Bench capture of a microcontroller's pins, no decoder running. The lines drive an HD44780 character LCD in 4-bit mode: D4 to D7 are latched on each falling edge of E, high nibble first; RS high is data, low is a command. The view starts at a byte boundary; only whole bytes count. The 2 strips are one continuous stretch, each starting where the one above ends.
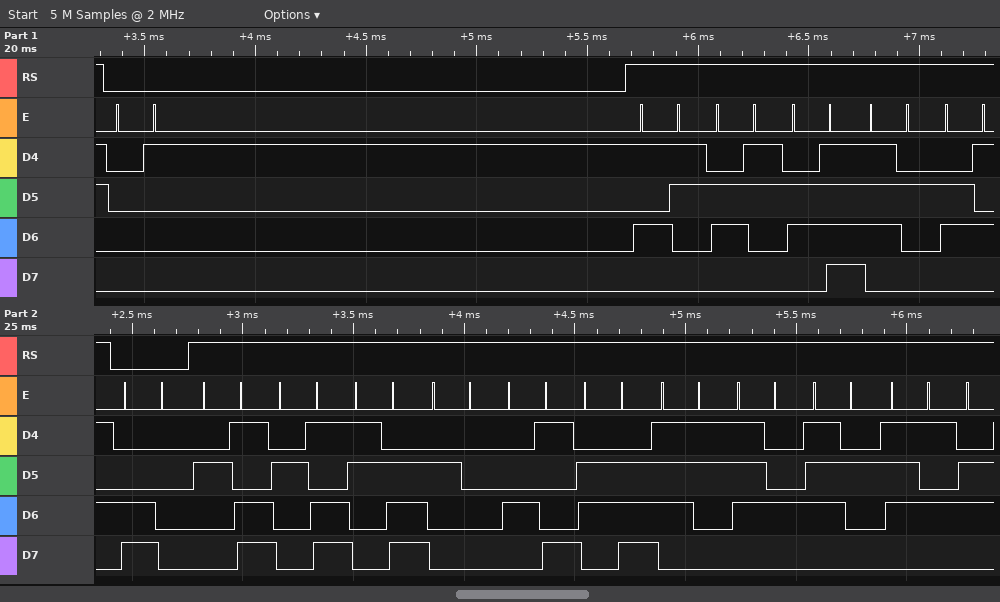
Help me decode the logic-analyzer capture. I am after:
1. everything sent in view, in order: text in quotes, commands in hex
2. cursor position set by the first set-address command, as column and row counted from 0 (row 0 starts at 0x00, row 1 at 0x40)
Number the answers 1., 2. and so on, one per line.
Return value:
1. 0x01 "Score" 0xC0 "--> Instru"
2. column 0, row 1
